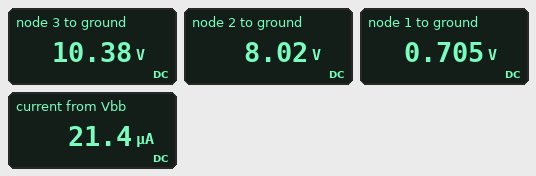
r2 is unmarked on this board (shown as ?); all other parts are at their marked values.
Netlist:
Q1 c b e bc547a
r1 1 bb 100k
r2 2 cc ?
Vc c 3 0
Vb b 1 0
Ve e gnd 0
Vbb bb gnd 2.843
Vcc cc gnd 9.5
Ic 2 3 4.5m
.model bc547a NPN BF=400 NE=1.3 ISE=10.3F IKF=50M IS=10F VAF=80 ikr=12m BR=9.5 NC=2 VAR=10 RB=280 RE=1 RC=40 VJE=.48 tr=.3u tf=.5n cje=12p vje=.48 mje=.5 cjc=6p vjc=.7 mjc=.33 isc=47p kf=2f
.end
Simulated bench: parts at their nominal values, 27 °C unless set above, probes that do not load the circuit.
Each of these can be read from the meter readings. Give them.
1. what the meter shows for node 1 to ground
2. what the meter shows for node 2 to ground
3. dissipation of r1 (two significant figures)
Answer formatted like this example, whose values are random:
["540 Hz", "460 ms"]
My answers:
["0.705 V", "8.02 V", "46 µW"]
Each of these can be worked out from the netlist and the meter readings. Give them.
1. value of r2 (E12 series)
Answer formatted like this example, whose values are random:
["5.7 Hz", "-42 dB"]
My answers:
["330 Ω"]
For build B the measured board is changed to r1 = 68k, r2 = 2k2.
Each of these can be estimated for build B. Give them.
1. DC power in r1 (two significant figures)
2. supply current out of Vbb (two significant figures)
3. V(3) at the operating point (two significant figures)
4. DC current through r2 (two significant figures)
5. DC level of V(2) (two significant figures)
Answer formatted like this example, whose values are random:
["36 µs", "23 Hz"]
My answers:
["67 µW", "31 µA", "310 mV", "4.5 mA", "-400 mV"]
